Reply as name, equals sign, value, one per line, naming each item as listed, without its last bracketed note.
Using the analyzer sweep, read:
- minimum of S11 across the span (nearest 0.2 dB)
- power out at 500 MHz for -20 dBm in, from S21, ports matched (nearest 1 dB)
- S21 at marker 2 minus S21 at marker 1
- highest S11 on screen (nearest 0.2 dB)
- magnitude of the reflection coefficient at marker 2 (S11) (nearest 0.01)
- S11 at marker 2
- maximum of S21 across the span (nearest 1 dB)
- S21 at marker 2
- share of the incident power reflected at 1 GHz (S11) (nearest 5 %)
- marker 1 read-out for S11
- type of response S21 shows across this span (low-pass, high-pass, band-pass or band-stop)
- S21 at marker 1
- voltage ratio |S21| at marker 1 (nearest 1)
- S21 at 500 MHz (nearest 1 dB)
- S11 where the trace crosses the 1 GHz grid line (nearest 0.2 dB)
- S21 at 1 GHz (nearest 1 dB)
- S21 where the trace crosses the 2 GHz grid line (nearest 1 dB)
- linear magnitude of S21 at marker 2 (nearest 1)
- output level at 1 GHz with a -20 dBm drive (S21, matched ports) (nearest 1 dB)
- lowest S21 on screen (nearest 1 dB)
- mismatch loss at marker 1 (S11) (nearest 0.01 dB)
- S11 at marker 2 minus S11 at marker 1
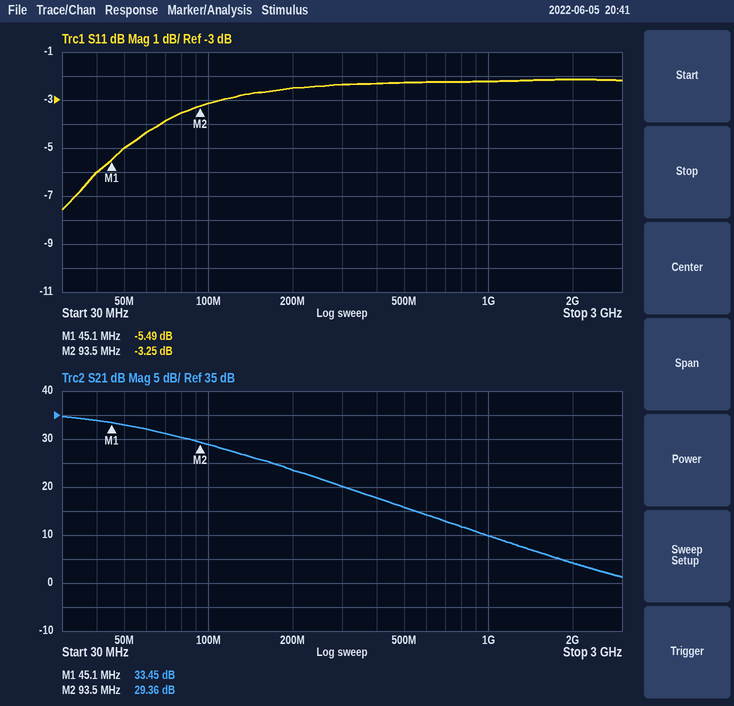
minimum of S11 across the span = -7.6 dB
power out at 500 MHz for -20 dBm in, from S21, ports matched = -4 dBm
S21 at marker 2 minus S21 at marker 1 = -4.09 dB
highest S11 on screen = -2.2 dB
magnitude of the reflection coefficient at marker 2 (S11) = 0.69
S11 at marker 2 = -3.25 dB
maximum of S21 across the span = 35 dB
S21 at marker 2 = 29.36 dB
share of the incident power reflected at 1 GHz (S11) = 60 %
marker 1 read-out for S11 = -5.49 dB
type of response S21 shows across this span = low-pass
S21 at marker 1 = 33.45 dB
voltage ratio |S21| at marker 1 = 47
S21 at 500 MHz = 16 dB
S11 where the trace crosses the 1 GHz grid line = -2.2 dB
S21 at 1 GHz = 10 dB
S21 where the trace crosses the 2 GHz grid line = 4 dB
linear magnitude of S21 at marker 2 = 29
output level at 1 GHz with a -20 dBm drive (S21, matched ports) = -10 dBm
lowest S21 on screen = 1 dB
mismatch loss at marker 1 (S11) = 1.44 dB
S11 at marker 2 minus S11 at marker 1 = 2.24 dB
